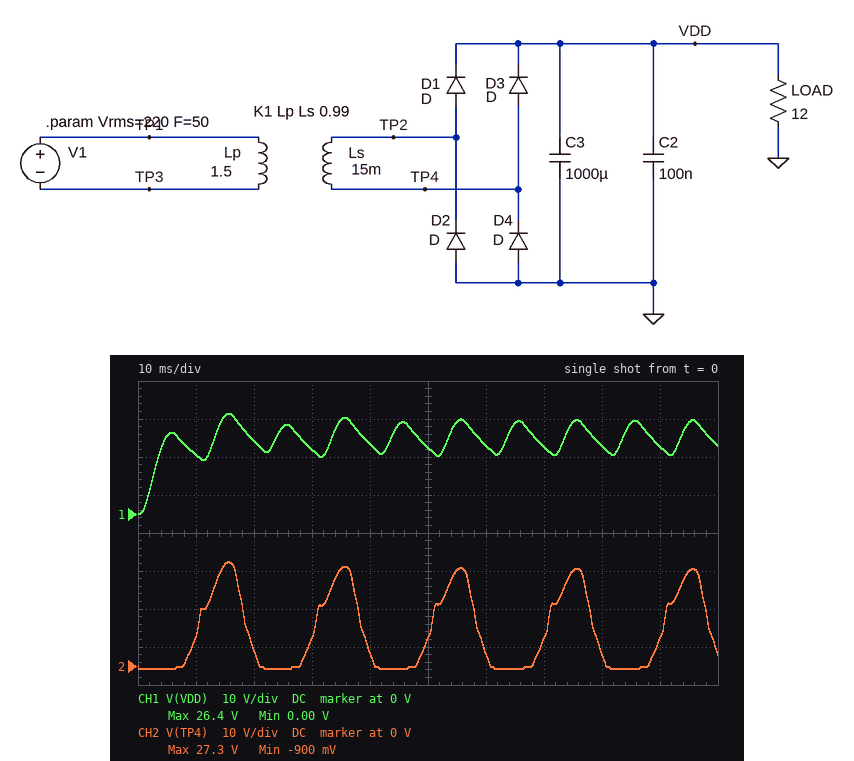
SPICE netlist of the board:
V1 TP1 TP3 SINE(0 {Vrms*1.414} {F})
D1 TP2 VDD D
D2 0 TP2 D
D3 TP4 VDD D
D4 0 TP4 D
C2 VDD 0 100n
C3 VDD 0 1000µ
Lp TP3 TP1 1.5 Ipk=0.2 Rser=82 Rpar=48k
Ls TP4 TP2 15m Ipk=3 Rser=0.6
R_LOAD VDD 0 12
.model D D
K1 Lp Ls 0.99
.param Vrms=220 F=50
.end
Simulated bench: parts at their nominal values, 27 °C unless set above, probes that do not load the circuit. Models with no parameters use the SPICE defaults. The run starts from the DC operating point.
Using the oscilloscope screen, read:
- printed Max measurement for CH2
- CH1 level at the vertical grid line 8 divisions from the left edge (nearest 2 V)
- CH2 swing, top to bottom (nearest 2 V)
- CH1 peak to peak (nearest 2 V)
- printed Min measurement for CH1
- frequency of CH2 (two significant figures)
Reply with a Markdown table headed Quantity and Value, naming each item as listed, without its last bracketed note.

| Quantity | Value |
|---|---|
| printed Max measurement for CH2 | 27.3 V |
| CH1 level at the vertical grid line 8 divisions from the left edge | 18 V |
| CH2 swing, top to bottom | 28 V |
| CH1 peak to peak | 26 V |
| printed Min measurement for CH1 | 0.00 V |
| frequency of CH2 | 50 Hz |
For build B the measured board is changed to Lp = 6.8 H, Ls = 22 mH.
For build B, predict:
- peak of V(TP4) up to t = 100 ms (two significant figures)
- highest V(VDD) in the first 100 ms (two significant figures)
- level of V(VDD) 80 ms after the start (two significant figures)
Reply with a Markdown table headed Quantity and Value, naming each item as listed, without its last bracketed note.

| Quantity | Value |
|---|---|
| peak of V(TP4) up to t = 100 ms | 16 V |
| highest V(VDD) in the first 100 ms | 15 V |
| level of V(VDD) 80 ms after the start | 11 V |
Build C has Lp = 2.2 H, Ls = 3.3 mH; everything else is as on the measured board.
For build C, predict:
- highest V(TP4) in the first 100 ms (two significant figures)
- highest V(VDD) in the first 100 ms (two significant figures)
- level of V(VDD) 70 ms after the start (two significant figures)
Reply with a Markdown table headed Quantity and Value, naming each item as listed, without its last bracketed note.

| Quantity | Value |
|---|---|
| highest V(TP4) in the first 100 ms | 11 V |
| highest V(VDD) in the first 100 ms | 10 V |
| level of V(VDD) 70 ms after the start | 6.5 V |
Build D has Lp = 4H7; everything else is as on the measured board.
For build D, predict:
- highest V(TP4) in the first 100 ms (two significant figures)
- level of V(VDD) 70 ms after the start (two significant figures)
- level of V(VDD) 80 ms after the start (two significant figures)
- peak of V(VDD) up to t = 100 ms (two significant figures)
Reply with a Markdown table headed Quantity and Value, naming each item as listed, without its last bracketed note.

| Quantity | Value |
|---|---|
| highest V(TP4) in the first 100 ms | 16 V |
| level of V(VDD) 70 ms after the start | 10 V |
| level of V(VDD) 80 ms after the start | 11 V |
| peak of V(VDD) up to t = 100 ms | 15 V |
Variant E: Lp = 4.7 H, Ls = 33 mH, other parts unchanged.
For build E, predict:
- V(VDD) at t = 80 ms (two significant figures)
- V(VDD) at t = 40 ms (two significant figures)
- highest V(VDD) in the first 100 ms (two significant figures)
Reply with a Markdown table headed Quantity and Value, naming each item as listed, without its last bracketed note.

| Quantity | Value |
|---|---|
| V(VDD) at t = 80 ms | 16 V |
| V(VDD) at t = 40 ms | 17 V |
| highest V(VDD) in the first 100 ms | 23 V |
